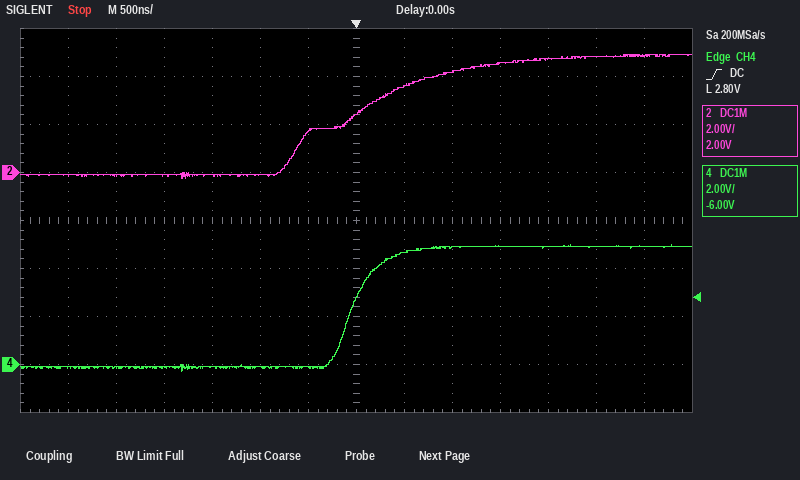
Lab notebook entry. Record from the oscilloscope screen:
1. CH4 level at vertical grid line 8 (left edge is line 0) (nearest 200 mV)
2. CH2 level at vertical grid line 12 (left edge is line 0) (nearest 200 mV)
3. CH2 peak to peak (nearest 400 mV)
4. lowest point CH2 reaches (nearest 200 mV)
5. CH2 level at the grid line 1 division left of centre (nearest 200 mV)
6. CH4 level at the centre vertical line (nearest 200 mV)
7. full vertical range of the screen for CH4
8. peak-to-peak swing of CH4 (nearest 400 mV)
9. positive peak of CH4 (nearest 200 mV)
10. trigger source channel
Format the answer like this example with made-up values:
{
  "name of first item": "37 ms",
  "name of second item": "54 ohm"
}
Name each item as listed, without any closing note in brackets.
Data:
{
  "CH4 level at vertical grid line 8 (left edge is line 0)": "4.6 V",
  "CH2 level at vertical grid line 12 (left edge is line 0)": "4.8 V",
  "CH2 peak to peak": "5.2 V",
  "lowest point CH2 reaches": "-200 mV",
  "CH2 level at the grid line 1 division left of centre": "1.8 V",
  "CH4 level at the centre vertical line": "2.8 V",
  "full vertical range of the screen for CH4": "16 V",
  "peak-to-peak swing of CH4": "5.2 V",
  "positive peak of CH4": "5.0 V",
  "trigger source channel": "CH4"
}
